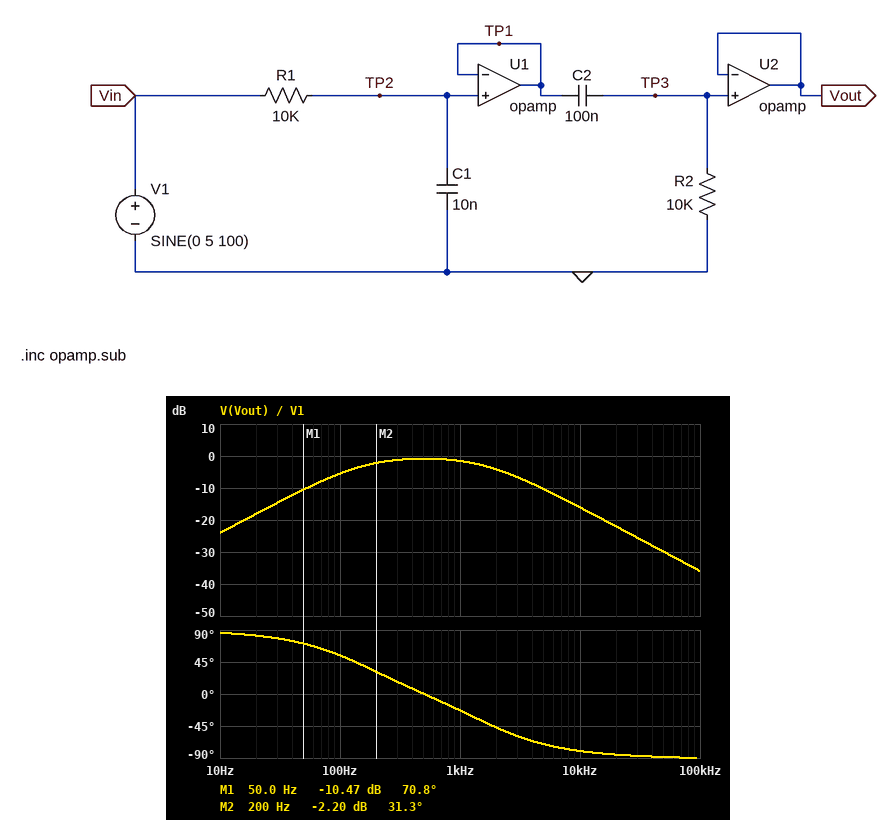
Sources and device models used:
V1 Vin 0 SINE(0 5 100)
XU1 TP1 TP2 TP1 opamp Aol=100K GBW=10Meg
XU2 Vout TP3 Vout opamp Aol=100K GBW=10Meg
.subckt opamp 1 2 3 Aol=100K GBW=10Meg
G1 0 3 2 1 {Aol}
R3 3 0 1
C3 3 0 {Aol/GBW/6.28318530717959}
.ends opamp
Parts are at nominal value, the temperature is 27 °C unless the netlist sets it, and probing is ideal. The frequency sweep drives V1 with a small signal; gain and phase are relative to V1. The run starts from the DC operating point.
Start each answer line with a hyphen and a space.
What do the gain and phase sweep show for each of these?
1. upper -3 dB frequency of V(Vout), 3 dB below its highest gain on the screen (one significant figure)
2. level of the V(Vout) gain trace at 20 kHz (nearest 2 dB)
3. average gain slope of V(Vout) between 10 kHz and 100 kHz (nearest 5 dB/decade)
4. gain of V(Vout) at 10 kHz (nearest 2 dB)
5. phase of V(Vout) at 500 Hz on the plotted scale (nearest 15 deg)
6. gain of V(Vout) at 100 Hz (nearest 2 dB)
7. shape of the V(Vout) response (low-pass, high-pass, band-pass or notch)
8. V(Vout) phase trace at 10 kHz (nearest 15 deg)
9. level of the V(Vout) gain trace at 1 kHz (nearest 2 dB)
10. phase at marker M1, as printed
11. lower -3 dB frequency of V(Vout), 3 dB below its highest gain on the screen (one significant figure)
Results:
- 2 kHz
- -22 dB
- -20 dB/decade
- -16 dB
- 0 deg
- -6 dB
- band-pass
- -75 deg
- -2 dB
- 70.8 deg
- 100 Hz
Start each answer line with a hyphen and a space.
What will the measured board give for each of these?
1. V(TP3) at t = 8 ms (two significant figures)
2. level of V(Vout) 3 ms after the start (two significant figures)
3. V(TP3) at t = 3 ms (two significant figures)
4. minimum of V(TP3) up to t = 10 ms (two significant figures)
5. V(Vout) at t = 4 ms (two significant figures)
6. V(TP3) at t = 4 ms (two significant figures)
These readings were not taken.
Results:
- -810 mV
- 680 mV
- 680 mV
- -2.7 V
- -880 mV
- -880 mV
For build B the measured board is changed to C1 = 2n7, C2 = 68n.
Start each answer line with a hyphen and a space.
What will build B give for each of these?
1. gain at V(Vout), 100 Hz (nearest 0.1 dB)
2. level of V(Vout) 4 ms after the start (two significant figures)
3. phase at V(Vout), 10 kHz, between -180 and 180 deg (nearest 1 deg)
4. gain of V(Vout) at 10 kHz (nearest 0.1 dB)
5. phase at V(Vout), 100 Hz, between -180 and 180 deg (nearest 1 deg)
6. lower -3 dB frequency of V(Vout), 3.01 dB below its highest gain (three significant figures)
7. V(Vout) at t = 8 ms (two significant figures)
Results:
- -8.1 dB
- -980 mV
- -58 deg
- -5.9 dB
- 66 deg
- 217 Hz
- -210 mV
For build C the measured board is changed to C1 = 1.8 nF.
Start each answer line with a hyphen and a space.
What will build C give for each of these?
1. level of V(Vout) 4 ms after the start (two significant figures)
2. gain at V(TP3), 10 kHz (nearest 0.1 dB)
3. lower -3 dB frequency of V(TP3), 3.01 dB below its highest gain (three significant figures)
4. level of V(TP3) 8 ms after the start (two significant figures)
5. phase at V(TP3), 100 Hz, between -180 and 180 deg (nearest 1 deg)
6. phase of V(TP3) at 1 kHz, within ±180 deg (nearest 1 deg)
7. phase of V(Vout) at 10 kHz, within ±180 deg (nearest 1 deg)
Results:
- -1.0 V
- -3.6 dB
- 154 Hz
- -680 mV
- 57 deg
- 3 deg
- -48 deg
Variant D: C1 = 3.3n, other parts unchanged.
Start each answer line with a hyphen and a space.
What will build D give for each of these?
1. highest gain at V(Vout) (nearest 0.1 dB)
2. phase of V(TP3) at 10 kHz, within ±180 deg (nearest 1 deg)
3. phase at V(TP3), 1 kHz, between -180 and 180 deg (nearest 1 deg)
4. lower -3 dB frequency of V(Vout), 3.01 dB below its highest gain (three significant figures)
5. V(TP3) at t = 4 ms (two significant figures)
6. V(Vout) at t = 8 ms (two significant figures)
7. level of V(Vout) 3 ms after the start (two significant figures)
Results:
- -0.3 dB
- -63 deg
- -3 deg
- 150 Hz
- -980 mV
- -700 mV
- 590 mV
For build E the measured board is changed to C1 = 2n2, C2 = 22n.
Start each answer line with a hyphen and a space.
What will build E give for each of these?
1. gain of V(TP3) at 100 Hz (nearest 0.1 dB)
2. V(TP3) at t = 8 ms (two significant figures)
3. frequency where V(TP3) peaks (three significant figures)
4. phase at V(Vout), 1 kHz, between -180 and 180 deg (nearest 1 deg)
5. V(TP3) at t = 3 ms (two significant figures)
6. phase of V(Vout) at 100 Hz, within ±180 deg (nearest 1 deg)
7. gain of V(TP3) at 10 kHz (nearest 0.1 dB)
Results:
- -17.3 dB
- 110 mV
- 2.29 kHz
- 28 deg
- -110 mV
- 81 deg
- -4.7 dB
